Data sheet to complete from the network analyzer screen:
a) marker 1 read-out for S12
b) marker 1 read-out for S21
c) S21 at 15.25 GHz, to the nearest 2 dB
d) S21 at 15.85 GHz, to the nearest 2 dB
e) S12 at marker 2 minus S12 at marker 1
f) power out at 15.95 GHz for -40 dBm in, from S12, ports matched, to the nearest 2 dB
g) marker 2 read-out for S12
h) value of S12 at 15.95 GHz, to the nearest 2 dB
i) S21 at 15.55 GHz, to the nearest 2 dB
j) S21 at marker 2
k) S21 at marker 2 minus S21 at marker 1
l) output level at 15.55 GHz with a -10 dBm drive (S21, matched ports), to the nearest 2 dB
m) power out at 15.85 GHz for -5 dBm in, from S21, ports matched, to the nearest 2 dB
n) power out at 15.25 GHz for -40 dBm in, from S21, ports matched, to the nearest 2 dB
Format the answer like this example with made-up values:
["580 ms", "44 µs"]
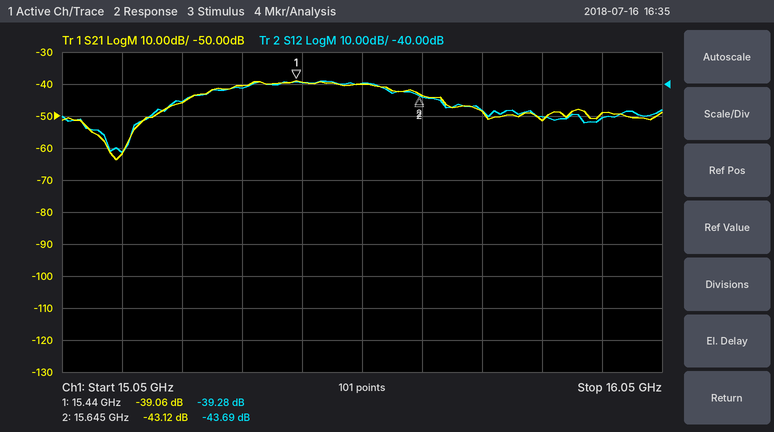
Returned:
["-39.28 dB", "-39.06 dB", "-46 dB", "-52 dB", "-4.41 dB", "-90 dBm", "-43.69 dB", "-50 dB", "-40 dB", "-43.12 dB", "-4.06 dB", "-50 dBm", "-56 dBm", "-86 dBm"]
